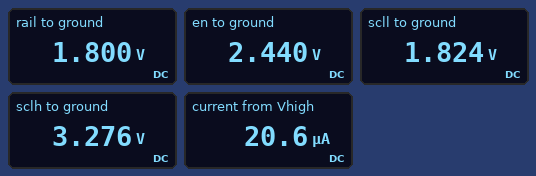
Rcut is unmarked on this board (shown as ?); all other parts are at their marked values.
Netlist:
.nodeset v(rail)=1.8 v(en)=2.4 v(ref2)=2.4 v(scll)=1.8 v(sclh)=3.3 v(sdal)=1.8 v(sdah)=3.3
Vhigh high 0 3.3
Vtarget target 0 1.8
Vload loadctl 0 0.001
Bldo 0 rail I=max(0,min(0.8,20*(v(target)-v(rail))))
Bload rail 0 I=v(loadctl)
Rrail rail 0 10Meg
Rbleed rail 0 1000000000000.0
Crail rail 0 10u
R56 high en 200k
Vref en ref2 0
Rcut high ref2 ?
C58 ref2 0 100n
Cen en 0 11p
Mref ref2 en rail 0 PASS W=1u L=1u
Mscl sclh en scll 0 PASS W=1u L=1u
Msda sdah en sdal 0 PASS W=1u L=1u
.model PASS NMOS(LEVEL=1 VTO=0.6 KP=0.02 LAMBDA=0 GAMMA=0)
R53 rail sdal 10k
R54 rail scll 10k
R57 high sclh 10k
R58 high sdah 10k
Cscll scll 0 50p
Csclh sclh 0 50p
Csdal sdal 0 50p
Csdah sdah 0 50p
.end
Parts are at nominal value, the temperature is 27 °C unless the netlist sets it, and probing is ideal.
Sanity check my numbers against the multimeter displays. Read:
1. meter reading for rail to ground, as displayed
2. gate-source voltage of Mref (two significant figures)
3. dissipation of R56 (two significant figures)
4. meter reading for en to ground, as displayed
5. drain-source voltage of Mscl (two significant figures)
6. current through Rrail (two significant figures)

1.800 V
640 mV
3.7 µW
2.440 V
1.5 V
180 nA
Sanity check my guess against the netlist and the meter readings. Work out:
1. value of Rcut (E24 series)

75 kΩ
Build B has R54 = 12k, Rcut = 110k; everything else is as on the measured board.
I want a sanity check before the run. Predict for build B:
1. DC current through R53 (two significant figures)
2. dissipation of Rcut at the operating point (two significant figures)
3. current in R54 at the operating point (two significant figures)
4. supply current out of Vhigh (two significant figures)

2.1 µA
6.8 µW
1.8 µA
16 µA
